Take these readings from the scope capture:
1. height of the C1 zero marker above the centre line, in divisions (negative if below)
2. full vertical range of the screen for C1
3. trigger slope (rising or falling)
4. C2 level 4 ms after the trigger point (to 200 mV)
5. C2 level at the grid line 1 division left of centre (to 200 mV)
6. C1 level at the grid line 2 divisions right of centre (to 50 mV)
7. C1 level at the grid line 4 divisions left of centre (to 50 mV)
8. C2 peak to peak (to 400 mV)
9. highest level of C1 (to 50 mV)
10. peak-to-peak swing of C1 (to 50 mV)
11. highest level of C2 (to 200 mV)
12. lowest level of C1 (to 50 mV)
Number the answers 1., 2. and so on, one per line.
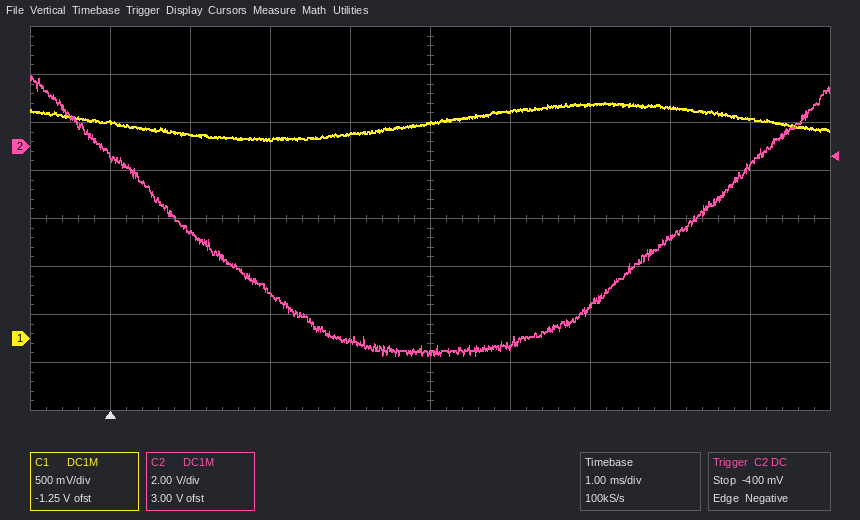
1. -2.5 div
2. 4 V
3. falling
4. -8.6 V
5. -8.0 V
6. 2.45 V
7. 2.25 V
8. 11.6 V
9. 2.45 V
10. 400 mV
11. 3.0 V
12. 2.05 V
